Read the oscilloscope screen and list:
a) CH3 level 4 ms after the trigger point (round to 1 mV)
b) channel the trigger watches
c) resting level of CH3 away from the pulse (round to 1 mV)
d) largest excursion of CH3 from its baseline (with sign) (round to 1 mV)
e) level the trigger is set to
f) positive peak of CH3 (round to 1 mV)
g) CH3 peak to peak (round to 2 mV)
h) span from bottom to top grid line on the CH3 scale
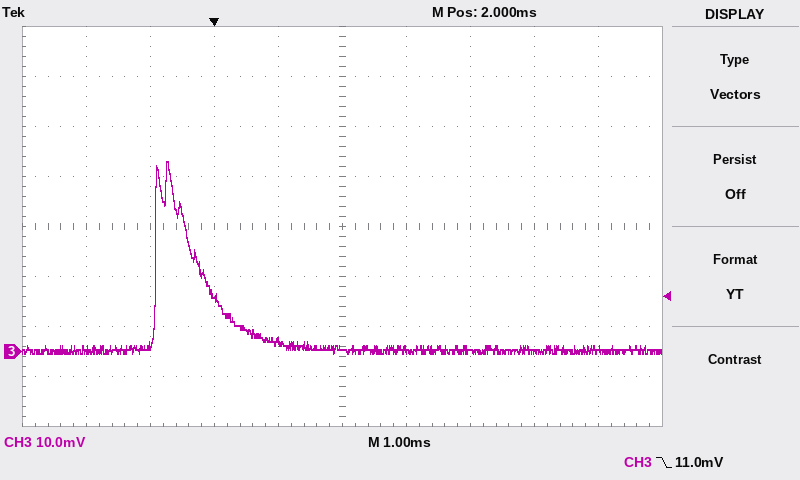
0 mV
CH3
0 mV
+38 mV
11.0 mV
38 mV
38 mV
80 mV
